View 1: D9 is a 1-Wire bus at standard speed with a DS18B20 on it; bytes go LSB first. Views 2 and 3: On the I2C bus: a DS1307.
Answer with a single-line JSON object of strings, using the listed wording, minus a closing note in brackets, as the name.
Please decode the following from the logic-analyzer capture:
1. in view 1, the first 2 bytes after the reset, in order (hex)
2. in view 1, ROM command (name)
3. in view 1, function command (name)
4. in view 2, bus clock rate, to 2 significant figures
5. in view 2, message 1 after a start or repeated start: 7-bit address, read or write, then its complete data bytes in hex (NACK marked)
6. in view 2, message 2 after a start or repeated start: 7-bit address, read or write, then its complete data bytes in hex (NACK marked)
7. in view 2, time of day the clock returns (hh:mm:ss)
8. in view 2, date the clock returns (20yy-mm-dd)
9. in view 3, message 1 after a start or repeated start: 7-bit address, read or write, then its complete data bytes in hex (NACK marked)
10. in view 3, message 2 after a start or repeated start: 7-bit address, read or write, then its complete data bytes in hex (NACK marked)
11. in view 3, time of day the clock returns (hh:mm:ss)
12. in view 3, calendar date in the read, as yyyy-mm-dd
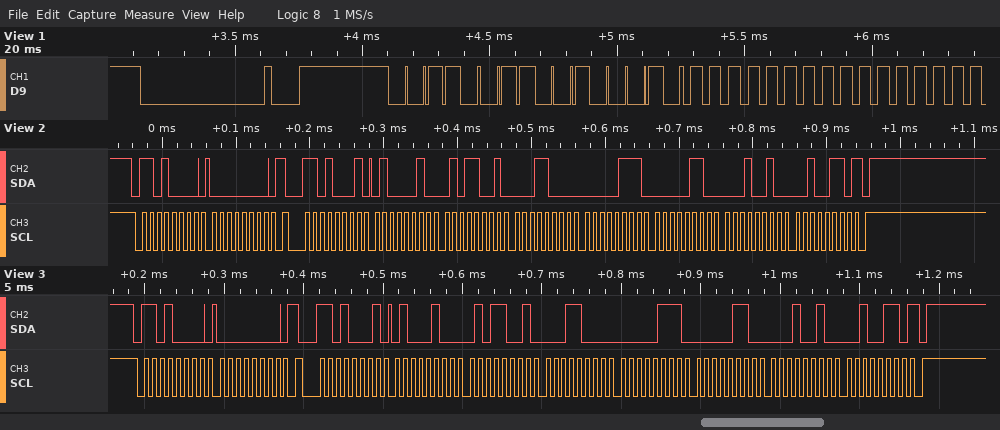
{"in view 1, the first 2 bytes after the reset, in order": "CC 44", "in view 1, ROM command": "Skip ROM", "in view 1, function command": "Convert T", "in view 2, bus clock rate, to 2 significant figures": "100 kHz", "in view 2, message 1 after a start or repeated start: 7-bit address, read or write, then its complete data bytes in hex": "0x68 write: 00", "in view 2, message 2 after a start or repeated start: 7-bit address, read or write, then its complete data bytes in hex": "0x68 read: 42 59 18 07 06 12 26 NACK", "in view 2, time of day the clock returns": "18:59:42", "in view 2, date the clock returns": "2026-12-06", "in view 3, message 1 after a start or repeated start: 7-bit address, read or write, then its complete data bytes in hex": "0x68 write: 00", "in view 3, message 2 after a start or repeated start: 7-bit address, read or write, then its complete data bytes in hex": "0x68 read: 44 59 18 07 06 12 26 NACK", "in view 3, time of day the clock returns": "18:59:44", "in view 3, calendar date in the read, as yyyy-mm-dd": "2026-12-06"}
